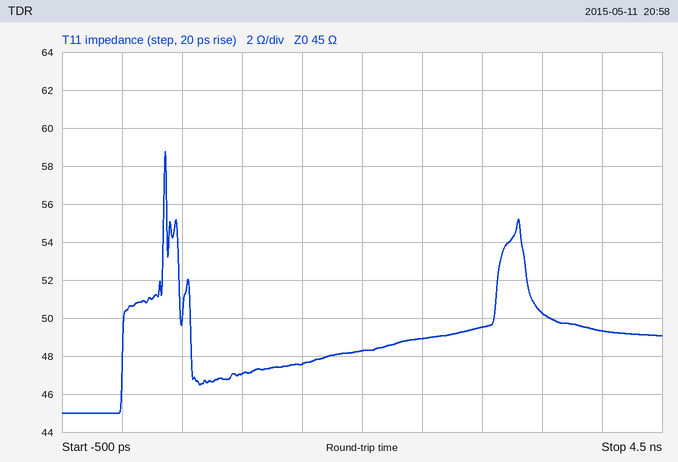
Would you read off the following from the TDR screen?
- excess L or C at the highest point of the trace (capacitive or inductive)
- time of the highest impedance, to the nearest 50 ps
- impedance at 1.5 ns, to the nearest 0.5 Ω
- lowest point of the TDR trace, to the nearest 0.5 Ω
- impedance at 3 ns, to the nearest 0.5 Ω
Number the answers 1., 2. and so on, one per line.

1. inductive
2. 350 ps
3. 47.5 Ω
4. 45.0 Ω
5. 49.5 Ω
